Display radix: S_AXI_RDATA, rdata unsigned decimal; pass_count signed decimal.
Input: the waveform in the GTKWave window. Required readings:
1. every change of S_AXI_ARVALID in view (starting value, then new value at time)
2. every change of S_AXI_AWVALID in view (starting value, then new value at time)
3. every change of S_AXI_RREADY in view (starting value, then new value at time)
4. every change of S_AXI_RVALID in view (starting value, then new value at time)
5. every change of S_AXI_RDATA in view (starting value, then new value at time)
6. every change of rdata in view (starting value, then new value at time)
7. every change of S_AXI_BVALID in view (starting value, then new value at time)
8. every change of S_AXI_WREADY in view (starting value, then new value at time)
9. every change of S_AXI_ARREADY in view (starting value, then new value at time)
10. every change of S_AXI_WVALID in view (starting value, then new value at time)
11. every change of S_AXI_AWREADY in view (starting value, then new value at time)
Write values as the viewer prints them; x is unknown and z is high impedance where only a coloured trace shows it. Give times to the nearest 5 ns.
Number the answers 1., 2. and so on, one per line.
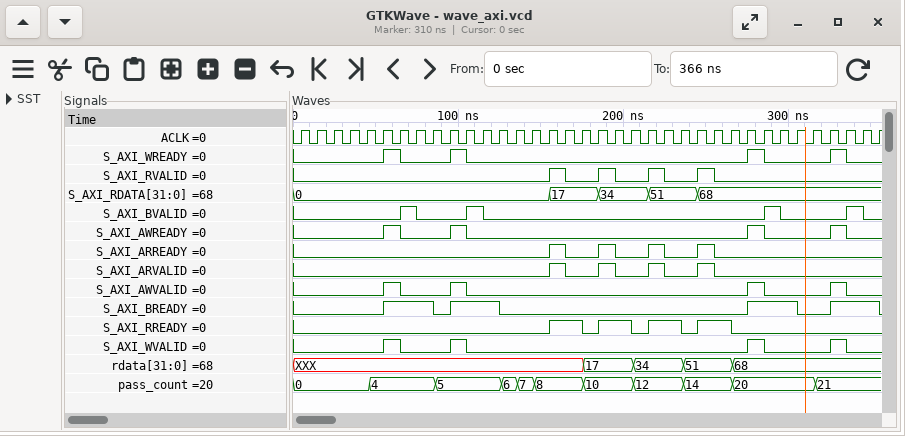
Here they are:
1. 0, 1 at 155 ns, 0 at 165 ns, 1 at 185 ns, 0 at 195 ns, 1 at 215 ns, 0 at 225 ns, 1 at 245 ns, 0 at 255 ns
2. 0, 1 at 55 ns, 0 at 65 ns, 1 at 95 ns, 0 at 105 ns, 1 at 275 ns, 0 at 285 ns, 1 at 325 ns, 0 at 335 ns
3. 0, 1 at 155 ns, 0 at 175 ns, 1 at 185 ns, 0 at 205 ns, 1 at 215 ns, 0 at 235 ns, 1 at 245 ns, 0 at 265 ns
4. 0, 1 at 155 ns, 0 at 165 ns, 1 at 185 ns, 0 at 195 ns, 1 at 215 ns, 0 at 225 ns, 1 at 245 ns, 0 at 255 ns
5. 0, 17 at 155 ns, 34 at 185 ns, 51 at 215 ns, 68 at 245 ns
6. XXX, 17 at 175 ns, 34 at 205 ns, 51 at 235 ns, 68 at 265 ns
7. 0, 1 at 65 ns, 0 at 75 ns, 1 at 105 ns, 0 at 115 ns, 1 at 285 ns, 0 at 295 ns, 1 at 335 ns, 0 at 345 ns
8. 0, 1 at 55 ns, 0 at 65 ns, 1 at 95 ns, 0 at 105 ns, 1 at 275 ns, 0 at 285 ns, 1 at 325 ns, 0 at 335 ns
9. 0, 1 at 155 ns, 0 at 165 ns, 1 at 185 ns, 0 at 195 ns, 1 at 215 ns, 0 at 225 ns, 1 at 245 ns, 0 at 255 ns
10. 0, 1 at 55 ns, 0 at 65 ns, 1 at 95 ns, 0 at 105 ns, 1 at 275 ns, 0 at 285 ns, 1 at 325 ns, 0 at 335 ns
11. 0, 1 at 55 ns, 0 at 65 ns, 1 at 95 ns, 0 at 105 ns, 1 at 275 ns, 0 at 285 ns, 1 at 325 ns, 0 at 335 ns
